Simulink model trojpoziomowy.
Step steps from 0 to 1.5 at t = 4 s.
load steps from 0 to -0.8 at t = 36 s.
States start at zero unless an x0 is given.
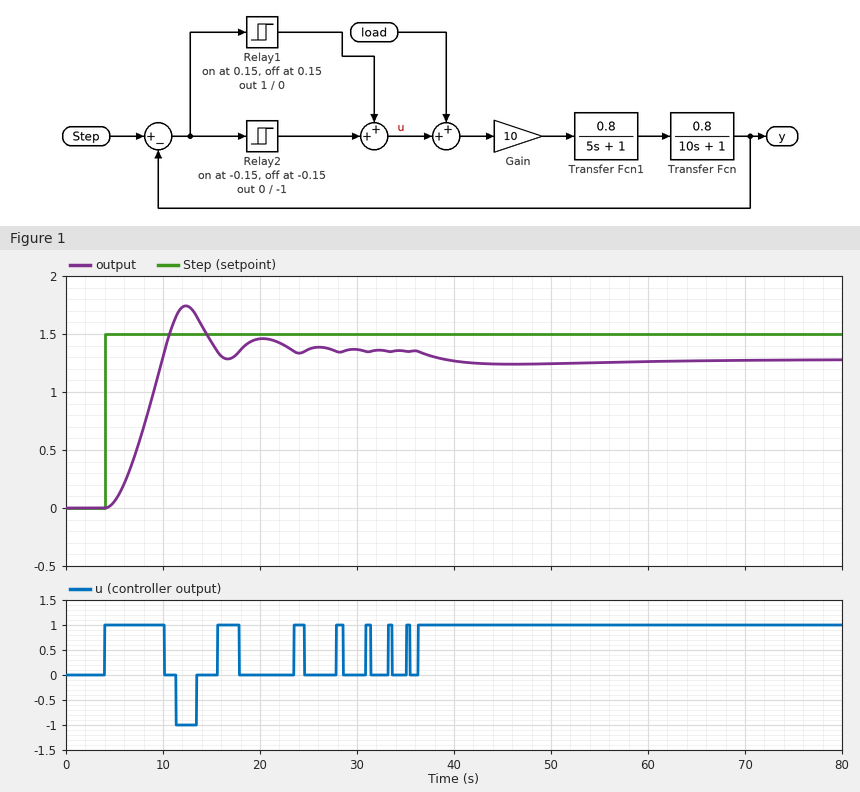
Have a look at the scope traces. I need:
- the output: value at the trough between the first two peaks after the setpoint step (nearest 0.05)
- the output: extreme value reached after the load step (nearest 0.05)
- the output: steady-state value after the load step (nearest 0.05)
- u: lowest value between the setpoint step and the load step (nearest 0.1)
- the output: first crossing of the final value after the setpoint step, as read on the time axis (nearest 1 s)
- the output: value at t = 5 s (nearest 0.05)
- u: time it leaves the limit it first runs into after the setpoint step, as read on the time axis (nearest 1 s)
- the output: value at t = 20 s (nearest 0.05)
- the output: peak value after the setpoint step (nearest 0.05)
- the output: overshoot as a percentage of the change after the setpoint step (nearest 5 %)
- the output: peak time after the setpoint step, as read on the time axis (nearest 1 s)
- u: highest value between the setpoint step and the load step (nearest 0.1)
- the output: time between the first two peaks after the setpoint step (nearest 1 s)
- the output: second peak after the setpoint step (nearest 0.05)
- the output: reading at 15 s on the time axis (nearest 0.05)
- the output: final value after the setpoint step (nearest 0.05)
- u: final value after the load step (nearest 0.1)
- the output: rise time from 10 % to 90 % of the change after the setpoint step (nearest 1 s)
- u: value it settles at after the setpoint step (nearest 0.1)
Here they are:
1.30
1.25
1.30
-1.0
10 s
0.05
10 s
1.45
1.75
30 %
12 s
1.0
8 s
1.45
1.45
1.35
1.0
4 s
0.0
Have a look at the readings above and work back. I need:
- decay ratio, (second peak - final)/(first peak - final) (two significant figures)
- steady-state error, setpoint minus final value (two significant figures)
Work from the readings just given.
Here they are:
0.25
0.15
